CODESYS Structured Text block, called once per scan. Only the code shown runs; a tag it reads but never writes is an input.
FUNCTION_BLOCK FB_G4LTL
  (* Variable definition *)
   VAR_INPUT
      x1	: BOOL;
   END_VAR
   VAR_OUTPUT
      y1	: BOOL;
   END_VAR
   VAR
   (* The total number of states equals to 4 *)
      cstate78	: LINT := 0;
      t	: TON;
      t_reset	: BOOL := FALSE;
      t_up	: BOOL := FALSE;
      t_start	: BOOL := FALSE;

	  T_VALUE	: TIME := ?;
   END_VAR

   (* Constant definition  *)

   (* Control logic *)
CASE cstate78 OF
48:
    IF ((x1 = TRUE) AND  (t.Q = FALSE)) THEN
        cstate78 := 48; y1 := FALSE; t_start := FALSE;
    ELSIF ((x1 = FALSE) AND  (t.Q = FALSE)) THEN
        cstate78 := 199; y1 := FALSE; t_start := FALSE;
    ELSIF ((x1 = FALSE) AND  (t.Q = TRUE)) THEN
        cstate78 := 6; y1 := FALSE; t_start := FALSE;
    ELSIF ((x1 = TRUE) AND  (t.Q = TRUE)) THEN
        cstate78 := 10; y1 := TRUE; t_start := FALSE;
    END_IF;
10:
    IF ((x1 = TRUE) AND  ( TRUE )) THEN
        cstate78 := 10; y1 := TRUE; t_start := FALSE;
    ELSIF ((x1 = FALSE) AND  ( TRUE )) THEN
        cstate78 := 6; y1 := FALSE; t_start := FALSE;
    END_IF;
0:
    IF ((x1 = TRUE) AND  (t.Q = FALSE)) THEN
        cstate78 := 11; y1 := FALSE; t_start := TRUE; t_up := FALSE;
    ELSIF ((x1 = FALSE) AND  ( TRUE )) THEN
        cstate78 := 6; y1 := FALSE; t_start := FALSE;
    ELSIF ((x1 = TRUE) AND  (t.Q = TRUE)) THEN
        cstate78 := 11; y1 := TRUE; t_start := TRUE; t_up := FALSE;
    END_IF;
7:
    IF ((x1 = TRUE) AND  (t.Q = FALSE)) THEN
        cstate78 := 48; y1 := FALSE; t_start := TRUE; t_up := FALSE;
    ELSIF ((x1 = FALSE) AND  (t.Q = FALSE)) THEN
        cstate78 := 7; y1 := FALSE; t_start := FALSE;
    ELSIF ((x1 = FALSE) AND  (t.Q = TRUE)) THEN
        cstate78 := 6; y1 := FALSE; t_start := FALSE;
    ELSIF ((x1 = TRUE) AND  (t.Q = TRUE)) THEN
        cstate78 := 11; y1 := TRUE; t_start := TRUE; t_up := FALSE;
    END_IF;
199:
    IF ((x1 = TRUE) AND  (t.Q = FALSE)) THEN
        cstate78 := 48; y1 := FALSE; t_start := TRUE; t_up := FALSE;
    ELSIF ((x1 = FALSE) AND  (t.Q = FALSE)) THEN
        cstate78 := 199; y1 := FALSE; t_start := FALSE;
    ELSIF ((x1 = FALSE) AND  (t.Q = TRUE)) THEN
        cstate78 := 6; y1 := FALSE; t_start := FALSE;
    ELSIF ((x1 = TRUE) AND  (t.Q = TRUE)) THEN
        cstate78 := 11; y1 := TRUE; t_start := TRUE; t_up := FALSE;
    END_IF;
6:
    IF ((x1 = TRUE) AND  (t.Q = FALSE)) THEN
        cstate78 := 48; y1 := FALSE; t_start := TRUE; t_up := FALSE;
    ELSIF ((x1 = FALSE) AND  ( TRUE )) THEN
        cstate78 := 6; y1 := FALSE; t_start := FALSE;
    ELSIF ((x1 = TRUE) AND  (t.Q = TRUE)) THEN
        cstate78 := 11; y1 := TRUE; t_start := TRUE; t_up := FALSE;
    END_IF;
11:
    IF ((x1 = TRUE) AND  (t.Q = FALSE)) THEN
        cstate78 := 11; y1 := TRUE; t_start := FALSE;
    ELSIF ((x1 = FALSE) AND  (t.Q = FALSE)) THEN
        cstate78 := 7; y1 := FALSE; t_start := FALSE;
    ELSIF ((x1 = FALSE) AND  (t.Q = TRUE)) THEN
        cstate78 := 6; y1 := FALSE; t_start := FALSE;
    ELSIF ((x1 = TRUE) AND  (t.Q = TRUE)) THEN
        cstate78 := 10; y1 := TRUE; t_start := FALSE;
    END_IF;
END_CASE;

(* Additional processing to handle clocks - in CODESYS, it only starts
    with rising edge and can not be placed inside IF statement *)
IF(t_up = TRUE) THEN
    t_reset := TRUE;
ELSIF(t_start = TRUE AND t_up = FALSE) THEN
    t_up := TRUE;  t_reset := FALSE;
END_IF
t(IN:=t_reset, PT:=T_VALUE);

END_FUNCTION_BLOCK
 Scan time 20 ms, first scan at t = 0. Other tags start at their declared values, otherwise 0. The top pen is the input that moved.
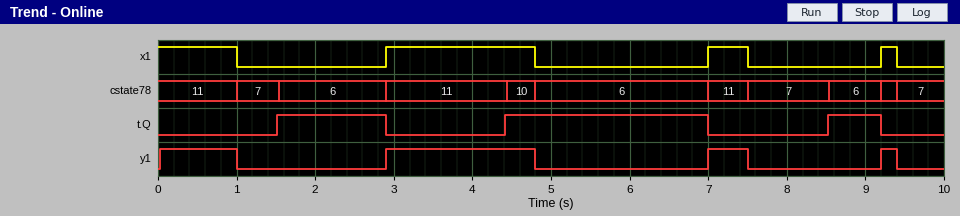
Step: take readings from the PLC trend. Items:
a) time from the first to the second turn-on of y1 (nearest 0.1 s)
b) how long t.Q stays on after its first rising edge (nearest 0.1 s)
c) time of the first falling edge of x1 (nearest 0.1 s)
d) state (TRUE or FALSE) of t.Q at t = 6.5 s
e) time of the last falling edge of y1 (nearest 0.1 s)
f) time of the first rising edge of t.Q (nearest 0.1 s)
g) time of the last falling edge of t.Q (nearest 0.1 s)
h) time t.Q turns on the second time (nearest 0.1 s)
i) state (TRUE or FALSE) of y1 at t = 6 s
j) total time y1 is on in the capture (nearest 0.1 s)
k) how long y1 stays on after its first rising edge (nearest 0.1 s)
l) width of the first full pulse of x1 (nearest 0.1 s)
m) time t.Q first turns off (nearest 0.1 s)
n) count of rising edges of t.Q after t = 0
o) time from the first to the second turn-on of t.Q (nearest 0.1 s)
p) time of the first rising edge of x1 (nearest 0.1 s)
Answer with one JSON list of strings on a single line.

["2.9 s", "1.4 s", "1.0 s", "TRUE", "9.4 s", "1.5 s", "9.2 s", "4.4 s", "FALSE", "3.6 s", "1.0 s", "1.9 s", "2.9 s", "3", "2.9 s", "2.9 s"]
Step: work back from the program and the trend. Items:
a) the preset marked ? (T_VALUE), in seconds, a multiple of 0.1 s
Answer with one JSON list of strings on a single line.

["1.5 s"]
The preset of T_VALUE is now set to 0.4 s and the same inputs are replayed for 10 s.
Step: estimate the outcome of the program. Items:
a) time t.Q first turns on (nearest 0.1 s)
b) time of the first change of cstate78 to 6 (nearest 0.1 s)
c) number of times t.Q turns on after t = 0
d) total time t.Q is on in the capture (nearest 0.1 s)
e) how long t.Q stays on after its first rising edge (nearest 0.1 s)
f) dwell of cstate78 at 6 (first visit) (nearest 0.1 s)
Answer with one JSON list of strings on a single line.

["0.4 s", "1.0 s", "4", "8.3 s", "2.5 s", "1.9 s"]
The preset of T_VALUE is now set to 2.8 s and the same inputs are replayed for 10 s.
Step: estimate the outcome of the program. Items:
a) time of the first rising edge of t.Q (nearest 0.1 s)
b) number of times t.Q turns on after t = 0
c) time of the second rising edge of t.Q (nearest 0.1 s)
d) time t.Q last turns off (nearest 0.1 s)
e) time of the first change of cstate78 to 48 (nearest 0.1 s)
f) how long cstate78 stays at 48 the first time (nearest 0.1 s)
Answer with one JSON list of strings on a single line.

["2.8 s", "2", "5.7 s", "7.0 s", "9.2 s", "0.2 s"]
